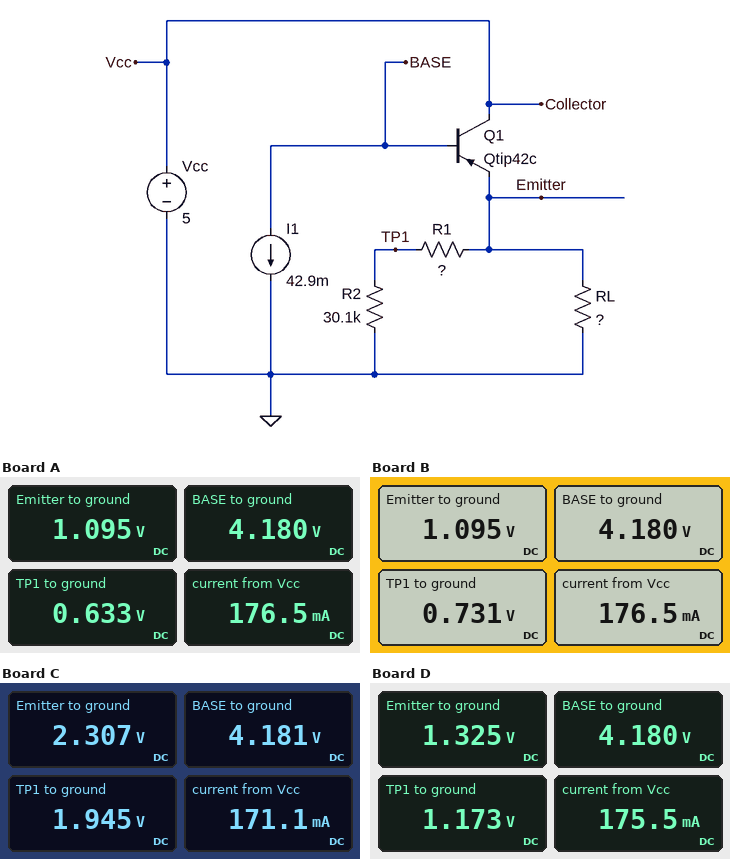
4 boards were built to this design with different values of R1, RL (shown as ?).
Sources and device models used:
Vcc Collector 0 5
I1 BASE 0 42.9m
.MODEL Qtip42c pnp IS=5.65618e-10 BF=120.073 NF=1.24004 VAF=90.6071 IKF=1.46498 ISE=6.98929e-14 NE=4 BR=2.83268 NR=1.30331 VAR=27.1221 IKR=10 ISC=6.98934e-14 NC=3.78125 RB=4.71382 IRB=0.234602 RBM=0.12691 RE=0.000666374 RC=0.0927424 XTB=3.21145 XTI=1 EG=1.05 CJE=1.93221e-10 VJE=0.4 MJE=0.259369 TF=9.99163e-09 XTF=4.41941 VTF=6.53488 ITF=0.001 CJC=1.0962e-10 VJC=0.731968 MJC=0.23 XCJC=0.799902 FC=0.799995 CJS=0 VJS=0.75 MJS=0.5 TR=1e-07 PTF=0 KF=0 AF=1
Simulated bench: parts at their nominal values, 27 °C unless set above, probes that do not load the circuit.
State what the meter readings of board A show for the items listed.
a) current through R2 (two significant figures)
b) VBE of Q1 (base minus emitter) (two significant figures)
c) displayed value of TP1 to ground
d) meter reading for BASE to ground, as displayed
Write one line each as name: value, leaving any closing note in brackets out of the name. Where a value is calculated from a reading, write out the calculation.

current through R2: (633 mV) / 30.1 kΩ = 21 µA
VBE of Q1 (base minus emitter): 4.18 V - 1.095 V = 3.1 V
displayed value of TP1 to ground: 0.633 V
meter reading for BASE to ground, as displayed: 4.180 V
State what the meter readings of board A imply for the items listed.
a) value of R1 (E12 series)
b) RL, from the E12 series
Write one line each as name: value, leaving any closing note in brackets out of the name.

value of R1: 22 kΩ
RL, from the E12 series: 8.2 Ω
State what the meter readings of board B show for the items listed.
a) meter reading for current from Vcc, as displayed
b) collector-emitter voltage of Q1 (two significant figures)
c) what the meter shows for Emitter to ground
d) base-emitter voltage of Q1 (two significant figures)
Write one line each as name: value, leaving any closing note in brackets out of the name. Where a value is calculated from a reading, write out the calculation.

meter reading for current from Vcc, as displayed: 176.5 mA
collector-emitter voltage of Q1: 5 V - 1.095 V = 3.9 V
what the meter shows for Emitter to ground: 1.095 V
base-emitter voltage of Q1: 4.18 V - 1.095 V = 3.1 V
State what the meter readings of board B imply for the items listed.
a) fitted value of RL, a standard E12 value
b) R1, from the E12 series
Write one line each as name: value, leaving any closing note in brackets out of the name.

fitted value of RL, a standard E12 value: 8.2 Ω
R1, from the E12 series: 15 kΩ
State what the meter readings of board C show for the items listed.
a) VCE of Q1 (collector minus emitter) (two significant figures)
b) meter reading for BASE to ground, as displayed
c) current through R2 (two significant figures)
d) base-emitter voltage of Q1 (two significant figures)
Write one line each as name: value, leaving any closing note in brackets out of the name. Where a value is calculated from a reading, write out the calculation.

VCE of Q1 (collector minus emitter): 5 V - 2.307 V = 2.7 V
meter reading for BASE to ground, as displayed: 4.181 V
current through R2: (1.945 V) / 30.1 kΩ = 65 µA
base-emitter voltage of Q1: 4.181 V - 2.307 V = 1.9 V
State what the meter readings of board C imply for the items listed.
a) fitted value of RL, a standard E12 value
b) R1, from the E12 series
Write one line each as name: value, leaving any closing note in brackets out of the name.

fitted value of RL, a standard E12 value: 18 Ω
R1, from the E12 series: 5.6 kΩ
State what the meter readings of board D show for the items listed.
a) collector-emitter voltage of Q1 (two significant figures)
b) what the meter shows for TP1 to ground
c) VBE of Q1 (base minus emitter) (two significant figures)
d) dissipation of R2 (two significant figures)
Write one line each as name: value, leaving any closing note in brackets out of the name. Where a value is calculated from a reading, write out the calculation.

collector-emitter voltage of Q1: 5 V - 1.325 V = 3.7 V
what the meter shows for TP1 to ground: 1.173 V
VBE of Q1 (base minus emitter): 4.18 V - 1.325 V = 2.9 V
dissipation of R2: (1.173 V)^2 / 30.1 kΩ = 46 µW
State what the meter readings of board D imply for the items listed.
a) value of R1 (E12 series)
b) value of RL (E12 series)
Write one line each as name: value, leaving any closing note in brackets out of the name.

value of R1: 3.9 kΩ
value of RL: 10 Ω
